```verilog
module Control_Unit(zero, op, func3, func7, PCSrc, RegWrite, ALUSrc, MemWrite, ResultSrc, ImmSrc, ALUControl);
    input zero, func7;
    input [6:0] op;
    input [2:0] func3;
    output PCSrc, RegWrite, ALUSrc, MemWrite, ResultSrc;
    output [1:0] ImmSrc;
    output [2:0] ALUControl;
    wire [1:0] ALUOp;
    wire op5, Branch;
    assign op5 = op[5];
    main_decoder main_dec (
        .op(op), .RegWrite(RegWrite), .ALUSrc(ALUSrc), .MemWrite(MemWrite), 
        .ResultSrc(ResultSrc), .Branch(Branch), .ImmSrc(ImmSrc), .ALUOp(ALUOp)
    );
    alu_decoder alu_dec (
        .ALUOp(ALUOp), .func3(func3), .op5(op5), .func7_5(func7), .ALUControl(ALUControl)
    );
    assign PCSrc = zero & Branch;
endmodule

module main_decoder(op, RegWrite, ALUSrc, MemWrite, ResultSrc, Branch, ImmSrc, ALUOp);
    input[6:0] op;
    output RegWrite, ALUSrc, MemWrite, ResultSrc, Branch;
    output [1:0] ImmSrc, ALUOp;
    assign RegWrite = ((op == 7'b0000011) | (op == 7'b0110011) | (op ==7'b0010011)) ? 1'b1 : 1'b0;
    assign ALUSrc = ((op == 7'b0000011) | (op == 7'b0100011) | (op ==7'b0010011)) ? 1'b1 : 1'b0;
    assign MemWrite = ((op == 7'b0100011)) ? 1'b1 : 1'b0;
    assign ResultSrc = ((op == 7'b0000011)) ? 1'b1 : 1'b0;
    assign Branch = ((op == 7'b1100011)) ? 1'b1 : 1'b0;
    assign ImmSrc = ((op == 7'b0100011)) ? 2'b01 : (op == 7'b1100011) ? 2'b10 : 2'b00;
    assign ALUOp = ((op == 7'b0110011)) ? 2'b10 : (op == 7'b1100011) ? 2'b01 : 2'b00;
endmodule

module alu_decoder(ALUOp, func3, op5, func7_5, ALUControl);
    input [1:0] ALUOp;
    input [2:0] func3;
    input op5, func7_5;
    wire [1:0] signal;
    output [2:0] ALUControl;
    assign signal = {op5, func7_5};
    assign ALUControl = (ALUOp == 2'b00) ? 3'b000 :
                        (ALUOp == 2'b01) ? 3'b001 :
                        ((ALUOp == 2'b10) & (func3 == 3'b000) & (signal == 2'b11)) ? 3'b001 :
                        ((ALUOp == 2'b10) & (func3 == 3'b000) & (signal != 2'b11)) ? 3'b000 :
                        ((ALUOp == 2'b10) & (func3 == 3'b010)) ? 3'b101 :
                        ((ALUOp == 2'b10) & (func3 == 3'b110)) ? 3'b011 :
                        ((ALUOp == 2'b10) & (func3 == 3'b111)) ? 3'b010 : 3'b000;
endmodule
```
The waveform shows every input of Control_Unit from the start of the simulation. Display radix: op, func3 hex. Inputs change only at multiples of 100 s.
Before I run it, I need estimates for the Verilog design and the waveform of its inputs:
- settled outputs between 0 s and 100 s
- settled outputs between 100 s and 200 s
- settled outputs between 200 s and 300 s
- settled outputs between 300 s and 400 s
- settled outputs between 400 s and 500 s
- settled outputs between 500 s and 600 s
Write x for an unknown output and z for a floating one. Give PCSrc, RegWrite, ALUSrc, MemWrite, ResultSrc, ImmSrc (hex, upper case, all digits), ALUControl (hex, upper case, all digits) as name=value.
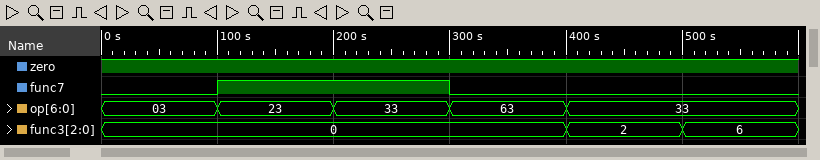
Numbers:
PCSrc=0, RegWrite=1, ALUSrc=1, MemWrite=0, ResultSrc=1, ImmSrc=0, ALUControl=0
PCSrc=0, RegWrite=0, ALUSrc=1, MemWrite=1, ResultSrc=0, ImmSrc=1, ALUControl=0
PCSrc=0, RegWrite=1, ALUSrc=0, MemWrite=0, ResultSrc=0, ImmSrc=0, ALUControl=1
PCSrc=1, RegWrite=0, ALUSrc=0, MemWrite=0, ResultSrc=0, ImmSrc=2, ALUControl=1
PCSrc=0, RegWrite=1, ALUSrc=0, MemWrite=0, ResultSrc=0, ImmSrc=0, ALUControl=5
PCSrc=0, RegWrite=1, ALUSrc=0, MemWrite=0, ResultSrc=0, ImmSrc=0, ALUControl=3
